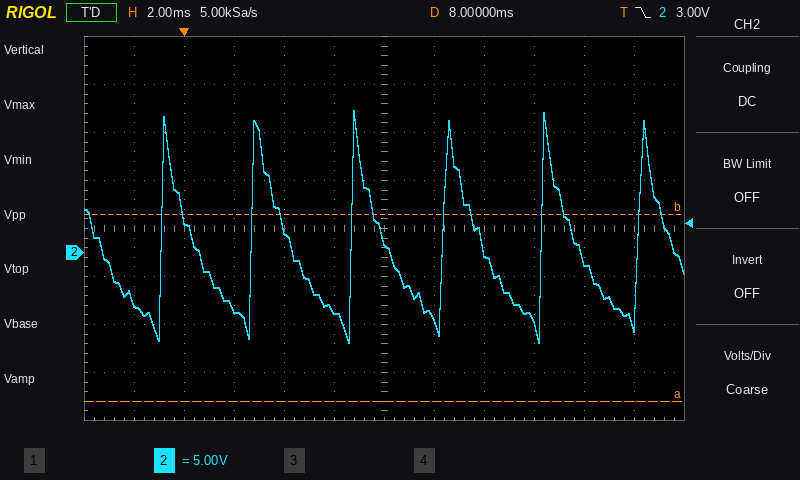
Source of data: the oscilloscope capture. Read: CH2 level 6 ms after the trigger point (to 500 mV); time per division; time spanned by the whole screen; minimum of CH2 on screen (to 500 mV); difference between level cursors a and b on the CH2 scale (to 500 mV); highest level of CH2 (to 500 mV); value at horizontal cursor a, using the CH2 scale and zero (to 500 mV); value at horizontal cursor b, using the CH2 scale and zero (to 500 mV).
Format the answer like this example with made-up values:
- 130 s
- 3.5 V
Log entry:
- -6.0 V
- 2 ms
- 24 ms
- -9.5 V
- 19.5 V
- 15.0 V
- -15.5 V
- 4.0 V
